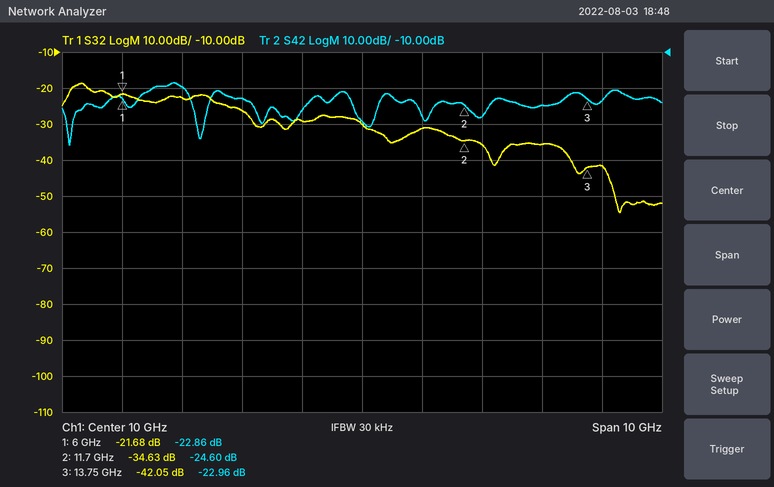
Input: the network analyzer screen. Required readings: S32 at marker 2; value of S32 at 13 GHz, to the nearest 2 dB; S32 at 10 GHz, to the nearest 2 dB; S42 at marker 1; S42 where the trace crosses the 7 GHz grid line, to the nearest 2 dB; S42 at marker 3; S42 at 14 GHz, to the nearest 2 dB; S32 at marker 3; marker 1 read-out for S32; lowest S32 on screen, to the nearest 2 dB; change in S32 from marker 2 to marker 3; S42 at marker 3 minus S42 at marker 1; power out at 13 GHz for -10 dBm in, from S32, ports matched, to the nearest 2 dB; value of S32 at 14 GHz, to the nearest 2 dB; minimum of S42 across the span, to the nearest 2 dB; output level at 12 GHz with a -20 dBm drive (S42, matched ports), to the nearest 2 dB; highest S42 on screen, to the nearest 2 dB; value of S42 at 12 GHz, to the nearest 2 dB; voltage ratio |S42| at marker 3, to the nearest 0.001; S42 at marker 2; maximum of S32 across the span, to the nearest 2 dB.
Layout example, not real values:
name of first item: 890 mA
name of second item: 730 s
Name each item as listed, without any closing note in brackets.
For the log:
S32 at marker 2: -34.63 dB
value of S32 at 13 GHz, to the nearest 2 dB: -36 dB
S32 at 10 GHz, to the nearest 2 dB: -30 dB
S42 at marker 1: -22.86 dB
S42 where the trace crosses the 7 GHz grid line, to the nearest 2 dB: -20 dB
S42 at marker 3: -22.96 dB
S42 at 14 GHz, to the nearest 2 dB: -24 dB
S32 at marker 3: -42.05 dB
marker 1 read-out for S32: -21.68 dB
lowest S32 on screen, to the nearest 2 dB: -54 dB
change in S32 from marker 2 to marker 3: -7.42 dB
S42 at marker 3 minus S42 at marker 1: -0.10 dB
power out at 13 GHz for -10 dBm in, from S32, ports matched, to the nearest 2 dB: -46 dBm
value of S32 at 14 GHz, to the nearest 2 dB: -42 dB
minimum of S42 across the span, to the nearest 2 dB: -36 dB
output level at 12 GHz with a -20 dBm drive (S42, matched ports), to the nearest 2 dB: -48 dBm
highest S42 on screen, to the nearest 2 dB: -18 dB
value of S42 at 12 GHz, to the nearest 2 dB: -28 dB
voltage ratio |S42| at marker 3, to the nearest 0.001: 0.071
S42 at marker 2: -24.60 dB
maximum of S32 across the span, to the nearest 2 dB: -18 dB
